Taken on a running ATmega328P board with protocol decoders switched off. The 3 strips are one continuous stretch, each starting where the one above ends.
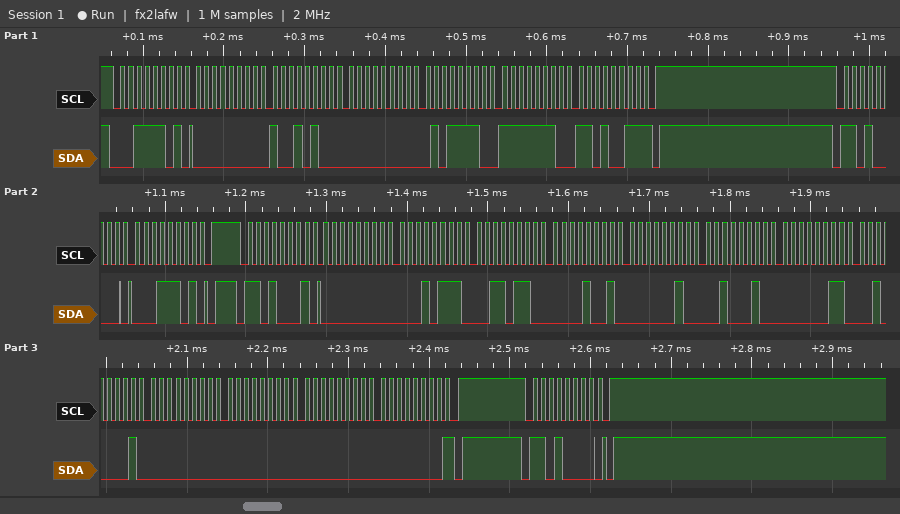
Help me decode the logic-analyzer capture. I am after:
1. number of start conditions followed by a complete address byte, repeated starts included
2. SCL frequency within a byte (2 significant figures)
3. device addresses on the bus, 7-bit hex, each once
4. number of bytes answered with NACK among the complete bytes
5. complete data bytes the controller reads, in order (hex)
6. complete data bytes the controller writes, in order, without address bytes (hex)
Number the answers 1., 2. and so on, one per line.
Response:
1. 4
2. 100 kHz
3. 0x1E 0x68
4. 2
5. 00 94 00 5E FE D3 00 17 36 09 02 22 03 21 00 00 00 00
6. 1D
